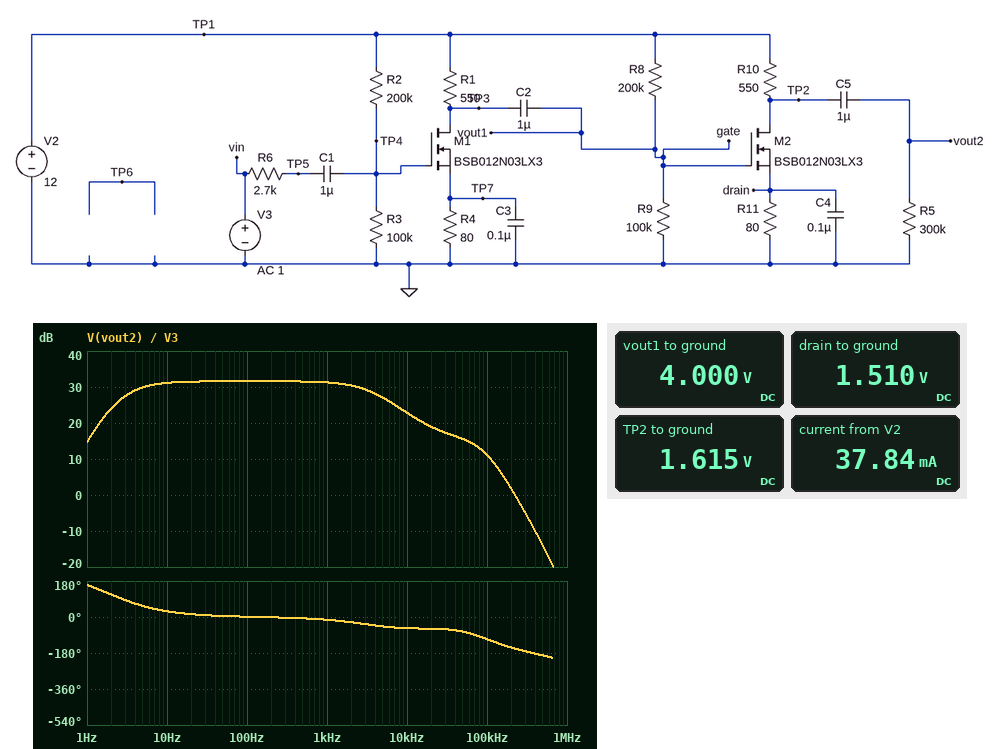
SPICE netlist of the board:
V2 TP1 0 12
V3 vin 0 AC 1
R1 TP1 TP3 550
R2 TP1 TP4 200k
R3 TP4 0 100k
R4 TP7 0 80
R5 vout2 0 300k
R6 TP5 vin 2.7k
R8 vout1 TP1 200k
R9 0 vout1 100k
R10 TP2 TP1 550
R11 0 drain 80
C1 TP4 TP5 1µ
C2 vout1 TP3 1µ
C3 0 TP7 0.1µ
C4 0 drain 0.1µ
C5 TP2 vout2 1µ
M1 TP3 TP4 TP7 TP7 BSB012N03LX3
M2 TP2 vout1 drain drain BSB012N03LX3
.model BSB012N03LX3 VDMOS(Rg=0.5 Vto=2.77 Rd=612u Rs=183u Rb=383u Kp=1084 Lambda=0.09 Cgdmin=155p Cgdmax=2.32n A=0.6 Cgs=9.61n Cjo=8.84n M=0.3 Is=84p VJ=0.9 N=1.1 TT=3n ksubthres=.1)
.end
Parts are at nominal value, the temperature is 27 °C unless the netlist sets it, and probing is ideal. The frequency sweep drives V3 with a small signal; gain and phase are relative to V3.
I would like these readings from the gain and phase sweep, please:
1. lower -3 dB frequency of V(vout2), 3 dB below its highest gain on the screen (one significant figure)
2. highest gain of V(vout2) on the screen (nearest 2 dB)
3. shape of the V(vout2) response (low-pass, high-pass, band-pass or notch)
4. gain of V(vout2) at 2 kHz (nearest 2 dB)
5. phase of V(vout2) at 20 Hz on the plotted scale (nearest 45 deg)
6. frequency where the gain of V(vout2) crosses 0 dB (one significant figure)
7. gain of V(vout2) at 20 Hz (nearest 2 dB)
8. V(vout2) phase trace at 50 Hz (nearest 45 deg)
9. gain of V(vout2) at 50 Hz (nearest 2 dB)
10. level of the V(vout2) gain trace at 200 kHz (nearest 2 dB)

4 Hz
32 dB
band-pass
30 dB
0 deg
200 kHz
32 dB
0 deg
32 dB
2 dB
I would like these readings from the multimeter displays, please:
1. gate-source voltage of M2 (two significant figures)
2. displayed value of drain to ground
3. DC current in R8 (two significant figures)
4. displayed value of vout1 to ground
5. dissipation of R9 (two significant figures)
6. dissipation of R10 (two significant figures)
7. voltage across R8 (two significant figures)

2.5 V
1.510 V
40 µA
4.000 V
160 µW
200 mW
8.0 V
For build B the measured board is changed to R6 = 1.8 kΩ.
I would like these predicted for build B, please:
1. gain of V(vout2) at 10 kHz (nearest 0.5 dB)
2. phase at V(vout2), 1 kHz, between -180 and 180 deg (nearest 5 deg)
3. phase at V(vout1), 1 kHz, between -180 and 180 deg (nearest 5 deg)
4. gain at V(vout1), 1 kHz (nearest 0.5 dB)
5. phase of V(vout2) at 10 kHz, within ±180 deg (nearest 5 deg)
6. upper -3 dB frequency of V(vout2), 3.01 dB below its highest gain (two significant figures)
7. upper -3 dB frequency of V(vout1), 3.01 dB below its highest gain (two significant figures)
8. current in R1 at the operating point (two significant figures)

25.5 dB
-10 deg
170 deg
15.5 dB
-50 deg
5.5 kHz
5.1 kHz
19 mA
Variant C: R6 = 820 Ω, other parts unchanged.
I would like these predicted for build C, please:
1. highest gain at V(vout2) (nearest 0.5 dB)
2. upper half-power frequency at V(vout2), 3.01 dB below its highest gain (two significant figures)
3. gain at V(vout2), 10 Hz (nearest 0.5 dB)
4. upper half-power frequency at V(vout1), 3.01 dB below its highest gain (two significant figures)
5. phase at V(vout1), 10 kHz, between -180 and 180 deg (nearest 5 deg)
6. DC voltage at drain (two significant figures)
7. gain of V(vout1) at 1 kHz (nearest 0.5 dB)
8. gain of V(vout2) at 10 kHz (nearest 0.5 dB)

32.0 dB
13 kHz
31.5 dB
10 kHz
130 deg
1.5 V
15.5 dB
30.0 dB
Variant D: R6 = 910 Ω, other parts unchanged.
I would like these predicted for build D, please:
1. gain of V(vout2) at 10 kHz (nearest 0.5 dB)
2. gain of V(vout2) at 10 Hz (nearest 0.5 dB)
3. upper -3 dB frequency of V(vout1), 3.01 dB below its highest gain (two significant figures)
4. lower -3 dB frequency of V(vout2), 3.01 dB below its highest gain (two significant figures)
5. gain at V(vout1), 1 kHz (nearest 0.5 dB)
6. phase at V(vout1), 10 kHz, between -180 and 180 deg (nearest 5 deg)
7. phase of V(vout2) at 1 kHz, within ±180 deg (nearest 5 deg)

29.5 dB
31.5 dB
9.4 kHz
3.7 Hz
15.5 dB
125 deg
-5 deg
